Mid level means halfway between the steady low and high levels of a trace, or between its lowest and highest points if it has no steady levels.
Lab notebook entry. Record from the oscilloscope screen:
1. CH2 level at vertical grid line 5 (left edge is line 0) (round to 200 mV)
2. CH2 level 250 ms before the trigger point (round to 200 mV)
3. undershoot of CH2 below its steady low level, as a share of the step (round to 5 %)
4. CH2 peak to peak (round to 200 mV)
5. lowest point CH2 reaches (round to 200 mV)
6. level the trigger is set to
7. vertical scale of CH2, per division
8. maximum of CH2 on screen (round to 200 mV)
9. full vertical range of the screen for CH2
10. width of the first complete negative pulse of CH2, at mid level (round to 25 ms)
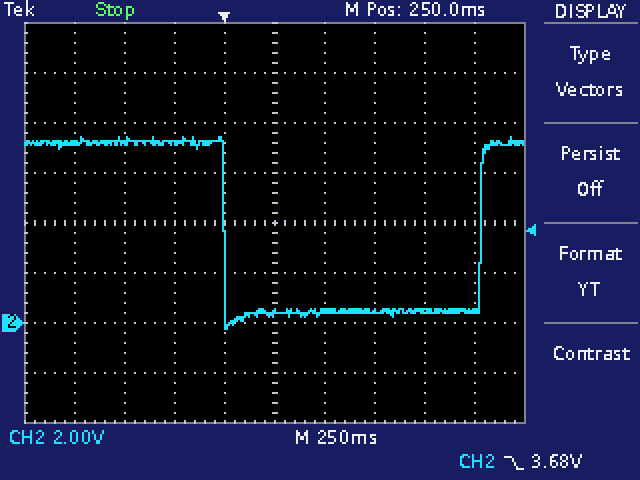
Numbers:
400 mV
7.2 V
10 %
7.6 V
-200 mV
3.68 V
2 V
7.4 V
16 V
1.275 s
